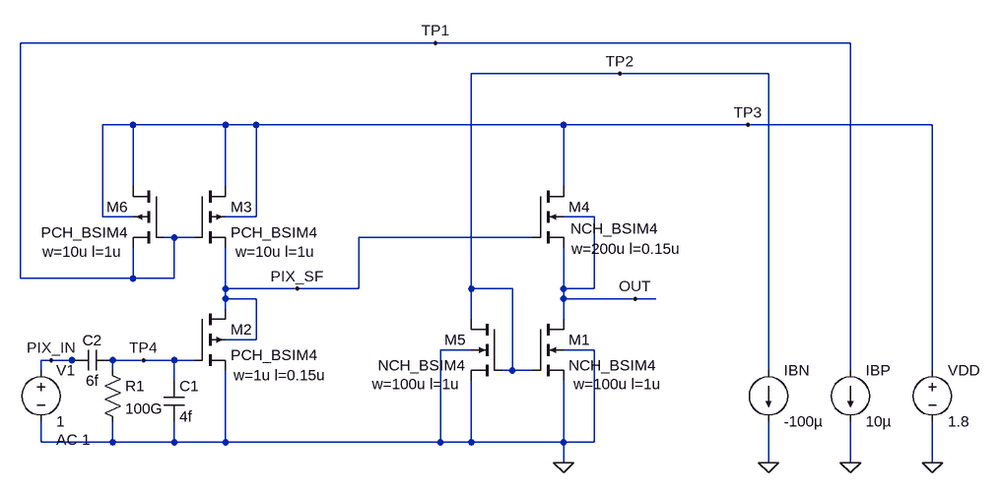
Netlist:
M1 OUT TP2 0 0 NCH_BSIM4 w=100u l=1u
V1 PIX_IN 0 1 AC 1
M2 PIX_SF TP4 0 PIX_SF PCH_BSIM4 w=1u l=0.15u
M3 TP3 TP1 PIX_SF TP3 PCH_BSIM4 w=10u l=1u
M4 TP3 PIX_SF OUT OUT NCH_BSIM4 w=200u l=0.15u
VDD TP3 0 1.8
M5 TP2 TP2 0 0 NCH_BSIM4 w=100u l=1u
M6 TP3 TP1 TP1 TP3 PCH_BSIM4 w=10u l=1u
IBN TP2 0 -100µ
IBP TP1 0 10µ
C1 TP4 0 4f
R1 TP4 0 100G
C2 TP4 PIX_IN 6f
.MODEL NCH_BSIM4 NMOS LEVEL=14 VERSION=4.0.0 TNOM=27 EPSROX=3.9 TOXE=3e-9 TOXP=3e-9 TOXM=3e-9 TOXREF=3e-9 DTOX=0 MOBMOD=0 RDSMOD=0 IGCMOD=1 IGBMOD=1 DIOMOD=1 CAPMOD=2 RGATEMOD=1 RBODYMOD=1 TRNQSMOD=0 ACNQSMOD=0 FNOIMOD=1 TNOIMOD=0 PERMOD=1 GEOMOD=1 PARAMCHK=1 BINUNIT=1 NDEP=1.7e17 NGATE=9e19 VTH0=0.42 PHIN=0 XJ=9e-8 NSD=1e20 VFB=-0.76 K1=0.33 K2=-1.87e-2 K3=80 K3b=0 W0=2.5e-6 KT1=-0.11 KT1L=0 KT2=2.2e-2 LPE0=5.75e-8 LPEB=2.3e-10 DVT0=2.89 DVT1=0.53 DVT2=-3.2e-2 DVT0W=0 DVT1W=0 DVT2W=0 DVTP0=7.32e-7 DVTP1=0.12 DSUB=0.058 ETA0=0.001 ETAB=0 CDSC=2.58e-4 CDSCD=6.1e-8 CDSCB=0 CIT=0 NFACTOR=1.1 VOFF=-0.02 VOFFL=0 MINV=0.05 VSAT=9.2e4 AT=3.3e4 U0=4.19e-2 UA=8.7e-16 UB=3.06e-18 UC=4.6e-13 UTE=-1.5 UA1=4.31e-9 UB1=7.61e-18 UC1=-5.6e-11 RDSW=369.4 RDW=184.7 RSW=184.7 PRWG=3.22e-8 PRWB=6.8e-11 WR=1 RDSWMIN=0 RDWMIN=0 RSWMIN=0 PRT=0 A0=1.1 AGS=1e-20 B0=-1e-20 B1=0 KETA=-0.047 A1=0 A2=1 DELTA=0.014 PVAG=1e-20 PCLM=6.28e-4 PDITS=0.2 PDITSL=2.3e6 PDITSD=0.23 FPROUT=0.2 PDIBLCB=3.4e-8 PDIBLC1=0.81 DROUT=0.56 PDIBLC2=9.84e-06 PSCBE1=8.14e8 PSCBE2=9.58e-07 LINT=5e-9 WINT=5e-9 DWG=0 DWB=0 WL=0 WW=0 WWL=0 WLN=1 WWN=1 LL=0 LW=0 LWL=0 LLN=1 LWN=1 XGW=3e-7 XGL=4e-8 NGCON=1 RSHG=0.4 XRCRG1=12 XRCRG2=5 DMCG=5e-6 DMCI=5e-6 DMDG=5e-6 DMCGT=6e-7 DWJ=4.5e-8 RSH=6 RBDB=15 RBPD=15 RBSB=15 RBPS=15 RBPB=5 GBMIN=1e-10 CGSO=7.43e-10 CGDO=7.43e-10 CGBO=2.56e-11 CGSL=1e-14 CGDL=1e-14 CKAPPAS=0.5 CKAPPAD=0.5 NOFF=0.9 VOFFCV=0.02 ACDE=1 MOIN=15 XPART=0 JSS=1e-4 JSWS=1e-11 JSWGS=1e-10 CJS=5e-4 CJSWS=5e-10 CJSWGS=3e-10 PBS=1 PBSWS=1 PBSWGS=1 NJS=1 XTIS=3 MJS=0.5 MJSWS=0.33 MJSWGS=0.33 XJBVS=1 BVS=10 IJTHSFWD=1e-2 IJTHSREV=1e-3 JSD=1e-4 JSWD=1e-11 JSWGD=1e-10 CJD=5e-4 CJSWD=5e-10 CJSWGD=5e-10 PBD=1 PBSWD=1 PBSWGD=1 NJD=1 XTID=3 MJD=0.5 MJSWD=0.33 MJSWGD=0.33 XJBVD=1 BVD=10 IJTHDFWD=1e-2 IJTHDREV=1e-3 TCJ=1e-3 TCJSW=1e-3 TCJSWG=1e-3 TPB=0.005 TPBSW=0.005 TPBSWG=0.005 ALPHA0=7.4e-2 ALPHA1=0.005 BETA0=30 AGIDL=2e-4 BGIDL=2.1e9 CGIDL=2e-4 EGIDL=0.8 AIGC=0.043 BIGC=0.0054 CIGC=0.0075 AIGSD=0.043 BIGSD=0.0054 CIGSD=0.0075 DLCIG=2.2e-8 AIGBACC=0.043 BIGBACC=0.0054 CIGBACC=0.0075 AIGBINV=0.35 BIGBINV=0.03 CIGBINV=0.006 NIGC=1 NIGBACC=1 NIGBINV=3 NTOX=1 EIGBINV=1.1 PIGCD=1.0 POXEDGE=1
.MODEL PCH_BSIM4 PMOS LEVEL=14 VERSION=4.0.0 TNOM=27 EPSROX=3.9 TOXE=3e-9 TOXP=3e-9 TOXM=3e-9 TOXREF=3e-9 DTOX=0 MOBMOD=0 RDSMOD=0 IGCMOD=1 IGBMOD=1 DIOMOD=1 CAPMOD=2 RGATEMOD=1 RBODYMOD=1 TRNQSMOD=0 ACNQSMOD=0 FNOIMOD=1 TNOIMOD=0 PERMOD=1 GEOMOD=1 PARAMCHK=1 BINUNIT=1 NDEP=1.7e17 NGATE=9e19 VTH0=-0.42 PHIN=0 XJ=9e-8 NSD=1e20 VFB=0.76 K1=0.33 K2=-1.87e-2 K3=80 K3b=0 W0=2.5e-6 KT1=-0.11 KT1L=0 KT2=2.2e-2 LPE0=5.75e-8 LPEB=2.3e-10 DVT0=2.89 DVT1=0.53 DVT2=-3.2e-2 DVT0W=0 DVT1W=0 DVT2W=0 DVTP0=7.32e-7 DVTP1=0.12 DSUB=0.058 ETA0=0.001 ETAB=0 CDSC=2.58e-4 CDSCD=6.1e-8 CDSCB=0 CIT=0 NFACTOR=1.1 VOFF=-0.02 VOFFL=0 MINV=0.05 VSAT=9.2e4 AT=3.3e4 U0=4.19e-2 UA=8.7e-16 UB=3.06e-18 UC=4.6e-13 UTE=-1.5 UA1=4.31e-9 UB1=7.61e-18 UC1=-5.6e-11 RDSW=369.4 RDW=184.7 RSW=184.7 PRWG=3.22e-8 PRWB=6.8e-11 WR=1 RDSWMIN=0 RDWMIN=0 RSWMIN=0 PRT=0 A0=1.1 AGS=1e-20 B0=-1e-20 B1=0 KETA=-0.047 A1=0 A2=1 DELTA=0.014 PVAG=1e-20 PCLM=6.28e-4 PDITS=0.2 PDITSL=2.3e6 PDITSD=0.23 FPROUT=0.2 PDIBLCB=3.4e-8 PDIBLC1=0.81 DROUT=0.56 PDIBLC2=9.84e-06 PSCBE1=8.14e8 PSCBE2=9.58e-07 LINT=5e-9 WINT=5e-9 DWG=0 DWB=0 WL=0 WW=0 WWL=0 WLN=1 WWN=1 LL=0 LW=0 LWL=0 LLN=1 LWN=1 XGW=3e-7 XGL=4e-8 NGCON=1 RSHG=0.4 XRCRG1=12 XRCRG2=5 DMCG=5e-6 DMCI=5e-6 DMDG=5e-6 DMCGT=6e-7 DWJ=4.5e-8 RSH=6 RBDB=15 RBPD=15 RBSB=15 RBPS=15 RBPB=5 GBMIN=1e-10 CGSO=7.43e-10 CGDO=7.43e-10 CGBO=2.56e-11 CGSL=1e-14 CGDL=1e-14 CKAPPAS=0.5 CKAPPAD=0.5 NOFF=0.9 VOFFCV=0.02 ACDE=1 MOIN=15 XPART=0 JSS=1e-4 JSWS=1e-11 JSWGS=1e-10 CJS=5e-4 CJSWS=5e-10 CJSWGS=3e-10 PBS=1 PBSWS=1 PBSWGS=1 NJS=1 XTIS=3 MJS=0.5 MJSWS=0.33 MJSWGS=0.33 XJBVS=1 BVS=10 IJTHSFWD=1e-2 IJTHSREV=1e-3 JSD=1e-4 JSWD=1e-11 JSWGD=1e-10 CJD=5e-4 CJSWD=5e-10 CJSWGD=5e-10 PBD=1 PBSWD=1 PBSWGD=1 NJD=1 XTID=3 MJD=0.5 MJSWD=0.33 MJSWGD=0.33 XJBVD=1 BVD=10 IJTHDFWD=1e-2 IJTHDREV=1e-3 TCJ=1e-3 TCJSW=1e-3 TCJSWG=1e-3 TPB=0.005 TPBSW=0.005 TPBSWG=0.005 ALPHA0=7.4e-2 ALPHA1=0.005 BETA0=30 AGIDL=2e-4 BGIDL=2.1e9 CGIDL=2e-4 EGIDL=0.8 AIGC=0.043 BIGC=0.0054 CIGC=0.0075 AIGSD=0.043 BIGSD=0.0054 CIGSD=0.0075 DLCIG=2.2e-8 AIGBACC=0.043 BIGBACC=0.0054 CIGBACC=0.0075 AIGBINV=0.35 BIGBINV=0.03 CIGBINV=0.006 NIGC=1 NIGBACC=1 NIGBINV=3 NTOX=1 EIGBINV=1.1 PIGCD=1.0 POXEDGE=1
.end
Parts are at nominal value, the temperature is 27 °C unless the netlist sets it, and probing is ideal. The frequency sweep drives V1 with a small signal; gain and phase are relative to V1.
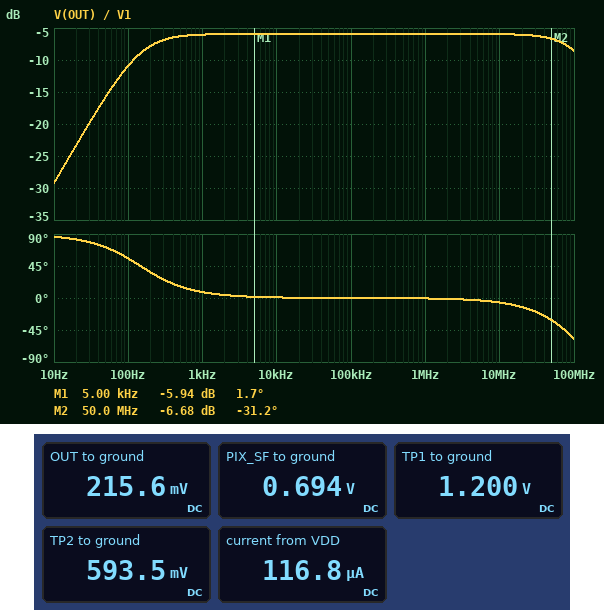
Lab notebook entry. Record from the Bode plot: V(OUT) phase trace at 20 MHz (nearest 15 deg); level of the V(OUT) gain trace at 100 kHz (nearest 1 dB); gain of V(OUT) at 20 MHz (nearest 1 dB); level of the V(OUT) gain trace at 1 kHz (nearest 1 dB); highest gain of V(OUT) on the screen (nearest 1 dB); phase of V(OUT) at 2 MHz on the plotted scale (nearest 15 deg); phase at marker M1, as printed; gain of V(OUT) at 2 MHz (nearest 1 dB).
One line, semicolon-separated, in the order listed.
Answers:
-15 deg; -6 dB; -6 dB; -6 dB; -6 dB; 0 deg; 1.7 deg; -6 dB
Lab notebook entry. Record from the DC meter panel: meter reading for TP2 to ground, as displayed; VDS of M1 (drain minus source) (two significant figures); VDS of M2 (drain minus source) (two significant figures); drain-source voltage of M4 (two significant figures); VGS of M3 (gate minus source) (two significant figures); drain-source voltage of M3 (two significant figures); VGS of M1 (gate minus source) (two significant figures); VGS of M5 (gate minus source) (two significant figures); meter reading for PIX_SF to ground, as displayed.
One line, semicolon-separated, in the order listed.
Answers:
593.5 mV; 220 mV; 690 mV; 1.6 V; 510 mV; 1.1 V; 590 mV; 590 mV; 0.694 V
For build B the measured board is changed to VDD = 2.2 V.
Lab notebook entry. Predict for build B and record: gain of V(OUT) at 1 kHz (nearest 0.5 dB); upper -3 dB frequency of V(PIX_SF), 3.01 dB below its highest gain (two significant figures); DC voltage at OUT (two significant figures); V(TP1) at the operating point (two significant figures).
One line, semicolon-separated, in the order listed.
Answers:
-6.5 dB; 110 MHz; 230 mV; 1.6 V
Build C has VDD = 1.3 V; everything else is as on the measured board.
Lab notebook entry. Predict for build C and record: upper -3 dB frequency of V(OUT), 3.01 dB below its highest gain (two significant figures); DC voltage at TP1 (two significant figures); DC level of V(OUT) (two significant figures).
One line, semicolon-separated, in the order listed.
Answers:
100 MHz; 700 mV; 200 mV
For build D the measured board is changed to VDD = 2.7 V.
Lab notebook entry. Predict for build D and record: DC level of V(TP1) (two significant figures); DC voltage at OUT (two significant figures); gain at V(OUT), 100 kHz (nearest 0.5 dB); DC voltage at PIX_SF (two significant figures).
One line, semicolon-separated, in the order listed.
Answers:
2.1 V; 290 mV; -7.0 dB; 700 mV
